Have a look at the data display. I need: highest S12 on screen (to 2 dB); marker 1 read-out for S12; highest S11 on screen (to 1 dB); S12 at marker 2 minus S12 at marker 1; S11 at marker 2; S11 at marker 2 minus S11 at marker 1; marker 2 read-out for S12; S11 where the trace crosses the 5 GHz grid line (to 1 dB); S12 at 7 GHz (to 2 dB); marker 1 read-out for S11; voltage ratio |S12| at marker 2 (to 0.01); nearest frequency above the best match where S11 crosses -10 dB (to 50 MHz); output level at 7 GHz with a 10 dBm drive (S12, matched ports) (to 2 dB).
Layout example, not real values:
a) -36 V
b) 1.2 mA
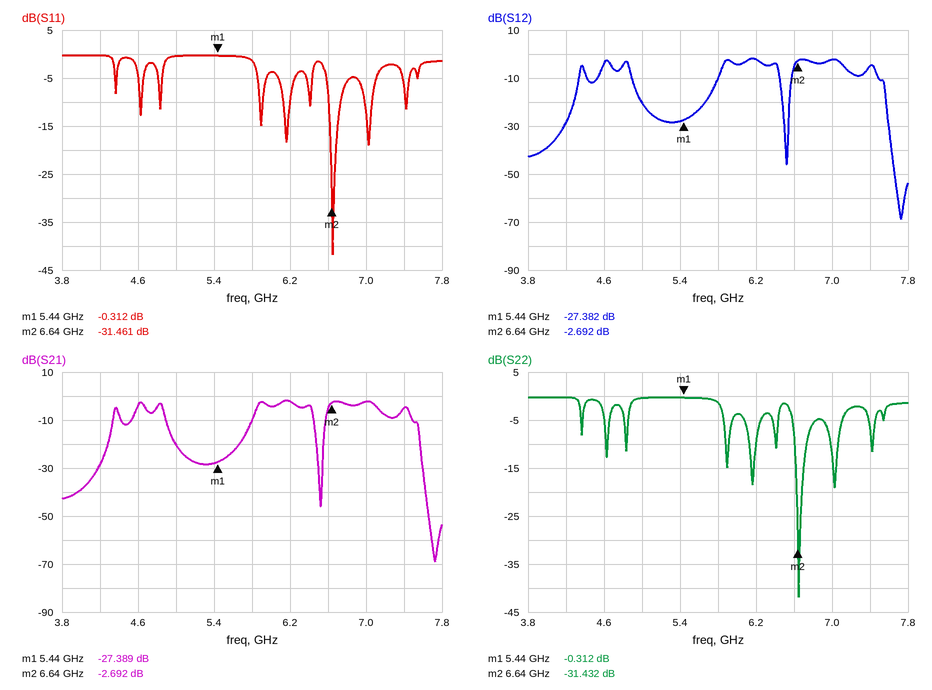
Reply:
a) -2 dB
b) -27.382 dB
c) 0 dB
d) 24.690 dB
e) -31.461 dB
f) -31.149 dB
g) -2.692 dB
h) 0 dB
i) -2 dB
j) -0.312 dB
k) 0.73
l) 6.75 GHz
m) 8 dBm
